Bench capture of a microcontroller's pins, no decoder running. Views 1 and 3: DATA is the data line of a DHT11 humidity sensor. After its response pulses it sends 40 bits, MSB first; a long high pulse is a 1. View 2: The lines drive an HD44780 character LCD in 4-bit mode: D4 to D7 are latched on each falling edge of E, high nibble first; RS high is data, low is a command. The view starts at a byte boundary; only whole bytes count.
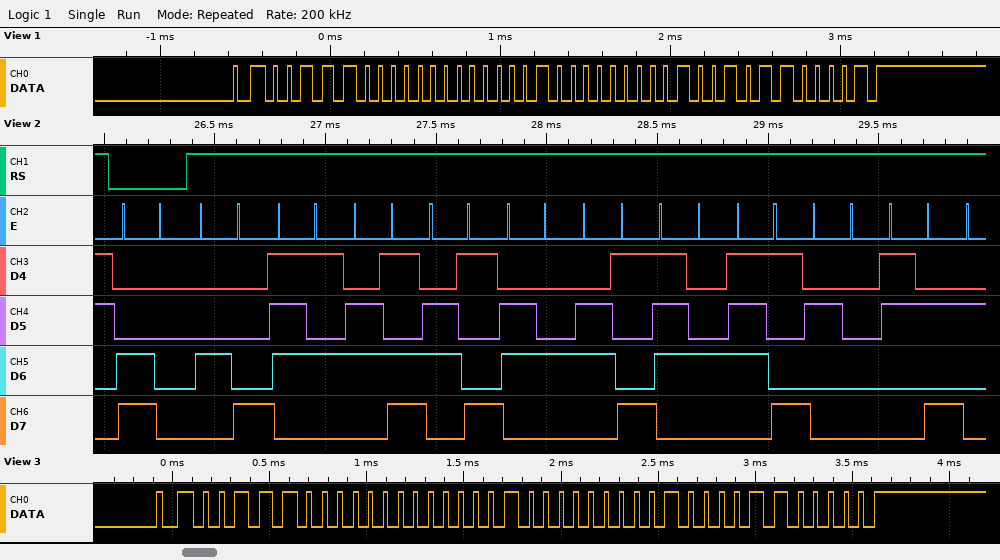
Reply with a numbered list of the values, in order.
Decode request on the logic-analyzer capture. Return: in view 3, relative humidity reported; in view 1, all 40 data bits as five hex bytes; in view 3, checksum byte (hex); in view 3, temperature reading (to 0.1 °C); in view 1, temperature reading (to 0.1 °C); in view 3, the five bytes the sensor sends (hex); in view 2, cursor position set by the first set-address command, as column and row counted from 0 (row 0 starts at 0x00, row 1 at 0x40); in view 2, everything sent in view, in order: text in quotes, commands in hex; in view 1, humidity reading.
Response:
1. 56 %
2. 38 00 20 09 61
3. 0x60
4. 32.8 °C
5. 32.9 °C
6. 38 00 20 08 60
7. column 0, row 1
8. 0xC0 "Humidity :"
9. 56 %
